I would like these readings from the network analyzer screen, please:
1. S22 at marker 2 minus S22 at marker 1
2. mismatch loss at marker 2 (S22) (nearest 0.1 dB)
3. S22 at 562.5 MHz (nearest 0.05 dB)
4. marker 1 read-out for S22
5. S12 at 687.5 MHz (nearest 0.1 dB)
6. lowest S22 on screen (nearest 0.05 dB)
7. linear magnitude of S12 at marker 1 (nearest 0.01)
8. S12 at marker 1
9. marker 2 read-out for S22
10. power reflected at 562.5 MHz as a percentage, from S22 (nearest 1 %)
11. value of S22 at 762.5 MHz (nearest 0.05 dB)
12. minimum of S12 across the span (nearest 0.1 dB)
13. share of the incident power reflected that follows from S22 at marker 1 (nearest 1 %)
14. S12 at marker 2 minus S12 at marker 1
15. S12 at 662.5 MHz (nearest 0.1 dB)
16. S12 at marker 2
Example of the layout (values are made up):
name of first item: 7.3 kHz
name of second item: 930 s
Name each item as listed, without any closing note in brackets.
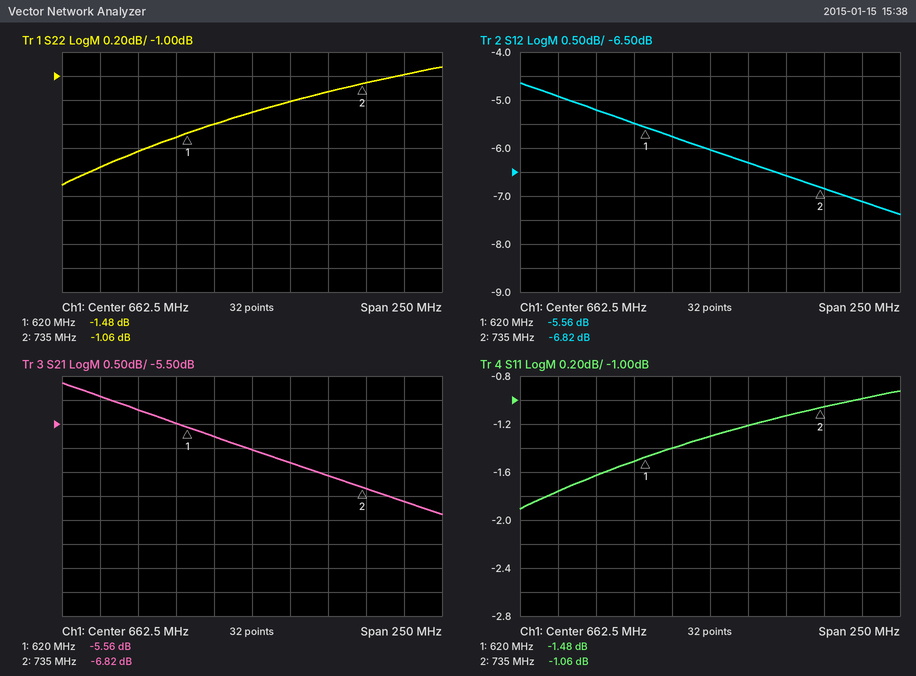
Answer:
S22 at marker 2 minus S22 at marker 1: 0.42 dB
mismatch loss at marker 2 (S22): 6.6 dB
S22 at 562.5 MHz: -1.75 dB
marker 1 read-out for S22: -1.48 dB
S12 at 687.5 MHz: -6.3 dB
lowest S22 on screen: -1.90 dB
linear magnitude of S12 at marker 1: 0.53
S12 at marker 1: -5.56 dB
marker 2 read-out for S22: -1.06 dB
power reflected at 562.5 MHz as a percentage, from S22: 67 %
value of S22 at 762.5 MHz: -1.00 dB
minimum of S12 across the span: -7.4 dB
share of the incident power reflected that follows from S22 at marker 1: 71 %
S12 at marker 2 minus S12 at marker 1: -1.26 dB
S12 at 662.5 MHz: -6.0 dB
S12 at marker 2: -6.82 dB
